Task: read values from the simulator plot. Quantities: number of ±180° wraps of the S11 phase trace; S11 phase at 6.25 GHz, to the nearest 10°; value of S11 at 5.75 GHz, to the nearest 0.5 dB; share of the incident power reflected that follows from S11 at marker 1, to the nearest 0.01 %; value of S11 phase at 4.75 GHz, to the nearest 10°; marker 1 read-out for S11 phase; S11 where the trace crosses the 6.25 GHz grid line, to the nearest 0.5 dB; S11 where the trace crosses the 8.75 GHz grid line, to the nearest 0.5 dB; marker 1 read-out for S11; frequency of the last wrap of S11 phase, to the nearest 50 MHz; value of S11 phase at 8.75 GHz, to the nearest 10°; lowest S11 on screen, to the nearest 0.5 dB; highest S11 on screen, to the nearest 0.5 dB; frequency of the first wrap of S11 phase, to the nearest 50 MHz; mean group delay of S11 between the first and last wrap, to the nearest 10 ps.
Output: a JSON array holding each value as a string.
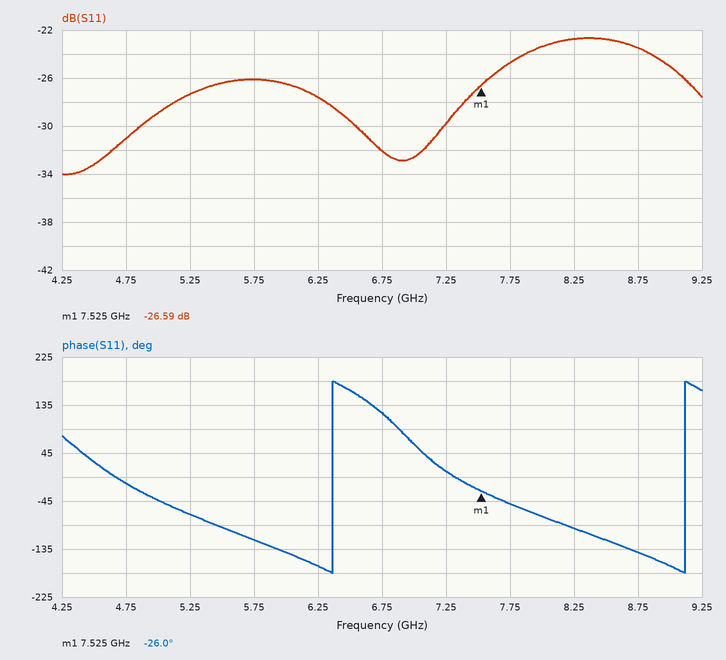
["2", "-170°", "-26.0 dB", "0.22 %", "-10°", "-26.0°", "-27.5 dB", "-23.5 dB", "-26.59 dB", "9.10 GHz", "-140°", "-34.0 dB", "-22.5 dB", "6.35 GHz", "360 ps"]
